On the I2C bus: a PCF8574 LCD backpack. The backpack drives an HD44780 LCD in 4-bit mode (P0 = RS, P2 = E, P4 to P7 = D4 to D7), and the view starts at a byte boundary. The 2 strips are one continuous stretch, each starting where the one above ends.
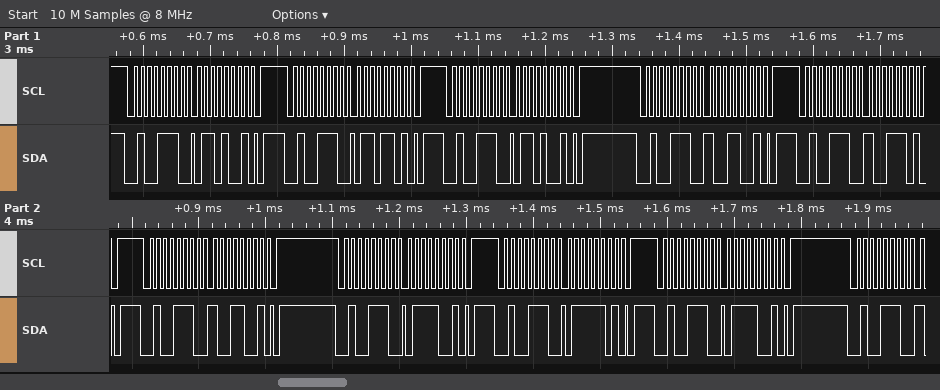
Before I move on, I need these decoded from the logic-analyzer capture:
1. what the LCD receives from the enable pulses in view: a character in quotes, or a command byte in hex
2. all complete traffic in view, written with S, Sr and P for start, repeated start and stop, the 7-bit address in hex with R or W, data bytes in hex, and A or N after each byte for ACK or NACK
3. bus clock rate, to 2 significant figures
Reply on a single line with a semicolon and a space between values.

'i'; S 27W A 69 A P S 27W A 6D A P S 27W A 69 A P S 27W A 99 A P S 27W A 9D A P S 27W A 99 A P S 27W A 79 A P S 27W A 7D A P S 27W A 79 A P S 27W A; 100 kHz
